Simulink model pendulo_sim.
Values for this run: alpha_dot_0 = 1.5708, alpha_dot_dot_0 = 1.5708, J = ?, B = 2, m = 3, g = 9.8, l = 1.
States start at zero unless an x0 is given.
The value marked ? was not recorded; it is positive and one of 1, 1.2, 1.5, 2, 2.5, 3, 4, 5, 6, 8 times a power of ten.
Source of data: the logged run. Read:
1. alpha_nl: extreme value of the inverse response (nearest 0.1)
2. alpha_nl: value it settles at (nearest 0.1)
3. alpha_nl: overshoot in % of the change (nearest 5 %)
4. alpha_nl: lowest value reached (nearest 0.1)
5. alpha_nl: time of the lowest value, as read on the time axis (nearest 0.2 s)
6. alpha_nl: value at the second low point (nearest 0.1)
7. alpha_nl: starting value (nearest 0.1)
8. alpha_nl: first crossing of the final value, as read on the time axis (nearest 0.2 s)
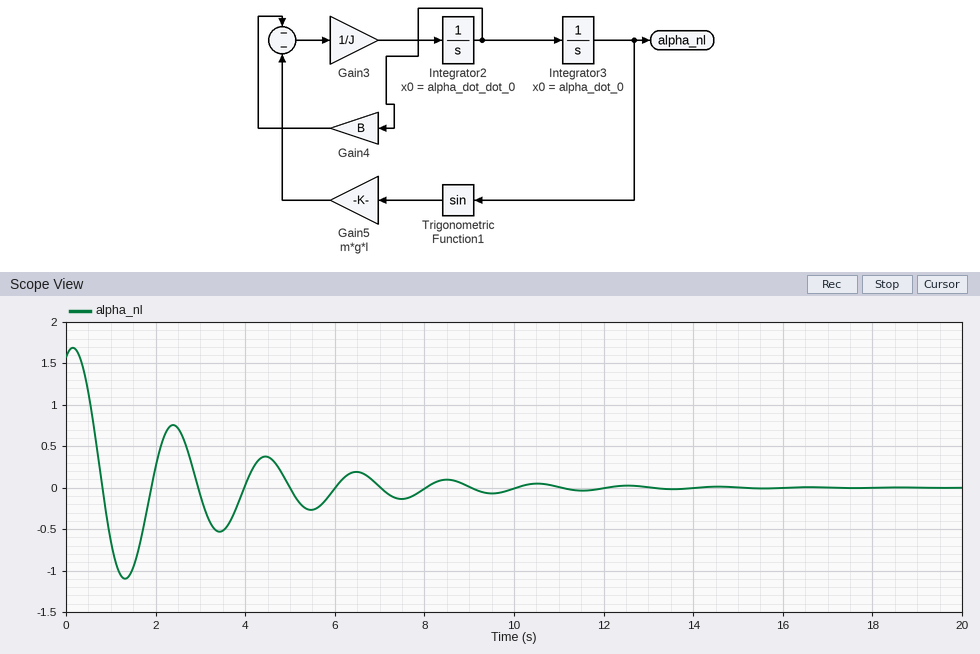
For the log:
1.7
0.0
70 %
-1.1
1.4 s
-0.5
1.6
0.8 s
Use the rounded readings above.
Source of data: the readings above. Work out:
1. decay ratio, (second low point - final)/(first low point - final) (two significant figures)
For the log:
0.45
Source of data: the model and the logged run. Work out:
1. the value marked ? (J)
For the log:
3
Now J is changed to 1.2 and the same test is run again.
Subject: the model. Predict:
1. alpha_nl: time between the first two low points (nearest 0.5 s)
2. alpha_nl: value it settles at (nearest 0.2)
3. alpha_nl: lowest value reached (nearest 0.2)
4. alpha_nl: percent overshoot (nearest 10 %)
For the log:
1.5 s
0.0
-0.8
50 %
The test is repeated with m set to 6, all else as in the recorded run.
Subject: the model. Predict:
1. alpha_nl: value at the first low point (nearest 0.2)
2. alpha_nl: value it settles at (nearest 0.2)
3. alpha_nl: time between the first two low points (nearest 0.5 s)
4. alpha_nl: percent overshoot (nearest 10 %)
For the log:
-1.2
0.0
1.5 s
80 %
